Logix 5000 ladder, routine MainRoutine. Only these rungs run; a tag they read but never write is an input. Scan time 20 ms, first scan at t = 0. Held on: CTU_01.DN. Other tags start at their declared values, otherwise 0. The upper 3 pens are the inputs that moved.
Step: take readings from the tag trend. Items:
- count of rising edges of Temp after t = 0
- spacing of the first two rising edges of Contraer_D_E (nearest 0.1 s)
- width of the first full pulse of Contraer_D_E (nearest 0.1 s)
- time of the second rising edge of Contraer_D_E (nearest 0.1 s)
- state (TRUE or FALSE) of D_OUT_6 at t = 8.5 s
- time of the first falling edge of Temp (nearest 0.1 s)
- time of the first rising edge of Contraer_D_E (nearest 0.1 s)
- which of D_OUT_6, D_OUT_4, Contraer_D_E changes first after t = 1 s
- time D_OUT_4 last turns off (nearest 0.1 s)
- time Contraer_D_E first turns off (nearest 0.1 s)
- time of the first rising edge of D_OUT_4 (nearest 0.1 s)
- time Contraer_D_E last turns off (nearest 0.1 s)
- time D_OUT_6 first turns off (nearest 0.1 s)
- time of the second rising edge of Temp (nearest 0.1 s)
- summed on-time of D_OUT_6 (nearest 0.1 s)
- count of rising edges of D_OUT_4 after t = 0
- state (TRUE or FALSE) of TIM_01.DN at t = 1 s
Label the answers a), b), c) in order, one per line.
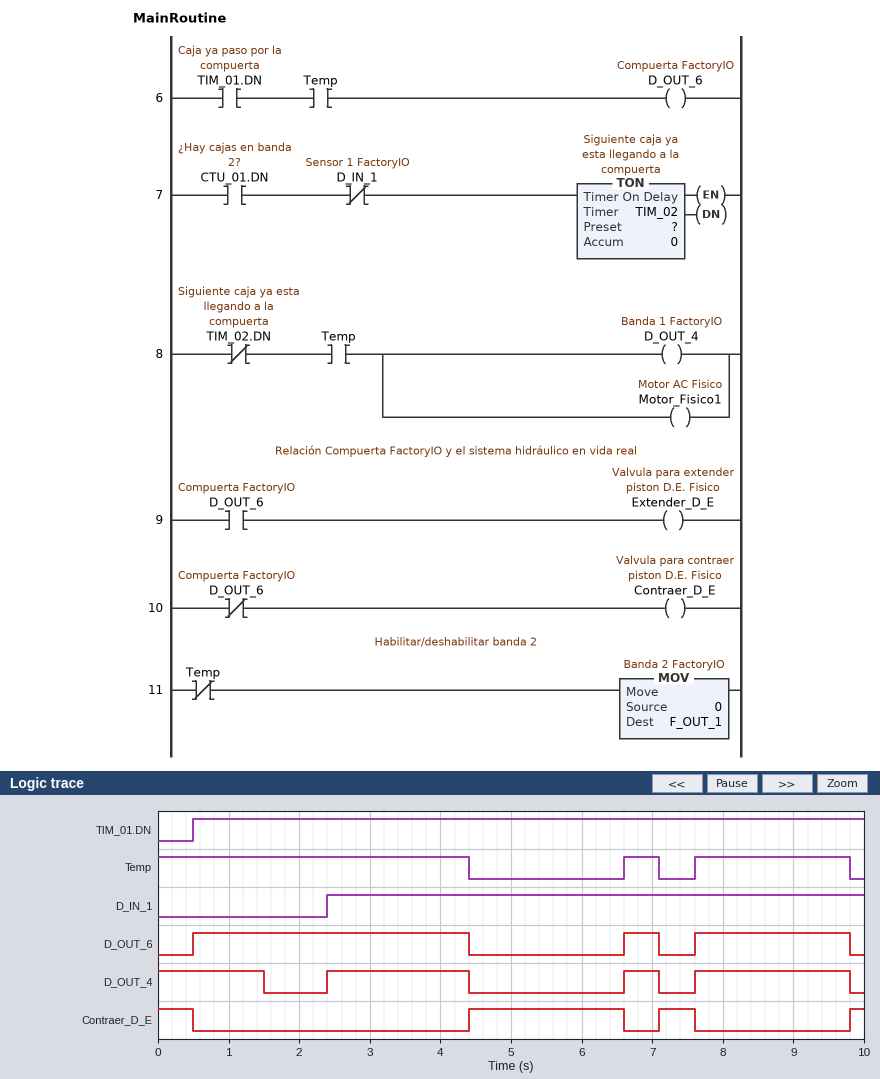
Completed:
a) 2
b) 2.7 s
c) 2.2 s
d) 7.1 s
e) TRUE
f) 4.4 s
g) 4.4 s
h) D_OUT_4
i) 9.8 s
j) 0.5 s
k) 2.4 s
l) 7.6 s
m) 4.4 s
n) 7.6 s
o) 6.6 s
p) 3
q) TRUE
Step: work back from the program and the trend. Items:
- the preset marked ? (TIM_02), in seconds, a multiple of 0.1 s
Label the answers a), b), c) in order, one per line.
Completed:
a) 1.5 s
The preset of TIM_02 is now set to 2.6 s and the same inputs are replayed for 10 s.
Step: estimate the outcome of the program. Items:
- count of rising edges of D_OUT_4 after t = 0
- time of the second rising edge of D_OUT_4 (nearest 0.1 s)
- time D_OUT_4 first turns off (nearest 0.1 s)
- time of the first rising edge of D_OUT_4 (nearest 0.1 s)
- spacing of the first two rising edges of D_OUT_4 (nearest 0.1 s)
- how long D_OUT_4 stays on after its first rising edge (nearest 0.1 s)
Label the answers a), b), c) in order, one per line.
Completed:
a) 2
b) 7.6 s
c) 4.4 s
d) 6.6 s
e) 1.0 s
f) 0.5 s
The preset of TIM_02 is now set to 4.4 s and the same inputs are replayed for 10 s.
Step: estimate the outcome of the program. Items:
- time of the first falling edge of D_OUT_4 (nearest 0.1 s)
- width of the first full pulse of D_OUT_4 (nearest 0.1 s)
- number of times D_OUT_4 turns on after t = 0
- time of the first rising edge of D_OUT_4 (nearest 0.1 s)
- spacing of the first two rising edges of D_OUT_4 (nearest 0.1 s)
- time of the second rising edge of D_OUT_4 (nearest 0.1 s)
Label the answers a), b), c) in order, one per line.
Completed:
a) 4.4 s
b) 0.5 s
c) 2
d) 6.6 s
e) 1.0 s
f) 7.6 s
